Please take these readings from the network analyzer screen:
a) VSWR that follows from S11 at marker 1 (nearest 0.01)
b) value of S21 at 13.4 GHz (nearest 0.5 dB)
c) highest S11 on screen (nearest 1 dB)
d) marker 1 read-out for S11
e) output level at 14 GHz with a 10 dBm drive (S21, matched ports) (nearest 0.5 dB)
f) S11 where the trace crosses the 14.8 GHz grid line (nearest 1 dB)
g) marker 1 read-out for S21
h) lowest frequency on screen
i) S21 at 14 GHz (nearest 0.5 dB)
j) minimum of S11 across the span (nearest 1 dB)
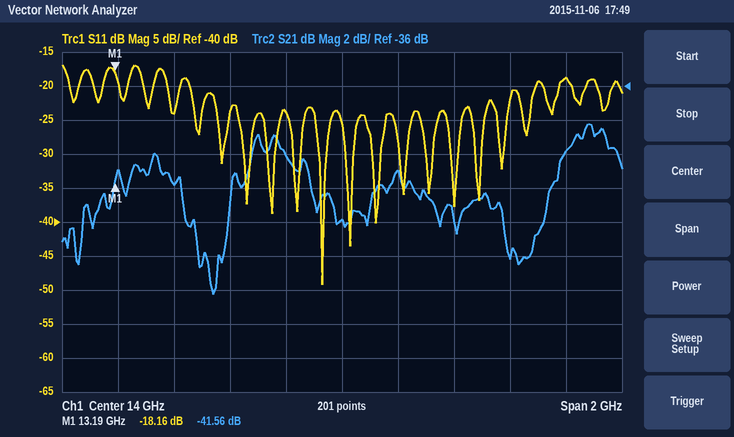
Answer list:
1.28
-42.0 dB
-17 dB
-18.16 dB
-34.0 dBm
-19 dB
-41.56 dB
13 GHz
-44.0 dB
-49 dB
